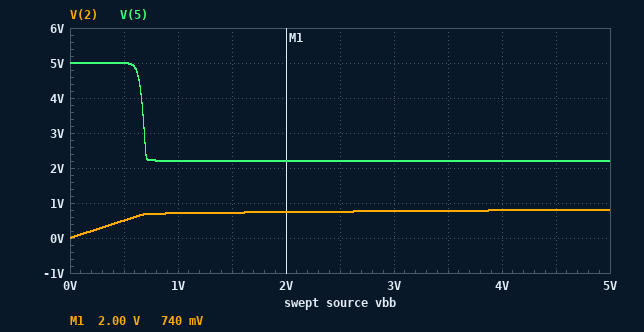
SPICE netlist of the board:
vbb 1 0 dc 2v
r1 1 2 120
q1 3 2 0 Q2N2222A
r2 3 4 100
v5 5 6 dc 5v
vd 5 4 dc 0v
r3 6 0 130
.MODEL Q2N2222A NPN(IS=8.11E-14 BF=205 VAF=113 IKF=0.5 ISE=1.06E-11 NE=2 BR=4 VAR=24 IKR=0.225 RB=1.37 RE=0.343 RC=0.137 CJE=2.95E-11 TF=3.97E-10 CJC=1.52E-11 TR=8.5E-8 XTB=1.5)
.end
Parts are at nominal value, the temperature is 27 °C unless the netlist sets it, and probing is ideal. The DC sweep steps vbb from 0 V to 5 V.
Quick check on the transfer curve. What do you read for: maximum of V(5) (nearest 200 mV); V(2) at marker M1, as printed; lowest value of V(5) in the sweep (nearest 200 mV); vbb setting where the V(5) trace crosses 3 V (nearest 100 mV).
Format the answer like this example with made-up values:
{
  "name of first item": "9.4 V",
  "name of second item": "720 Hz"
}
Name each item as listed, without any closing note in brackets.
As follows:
{
  "maximum of V(5)": "5.0 V",
  "V(2) at marker M1, as printed": "740 mV",
  "lowest value of V(5) in the sweep": "2.2 V",
  "vbb setting where the V(5) trace crosses 3 V": "700 mV"
}
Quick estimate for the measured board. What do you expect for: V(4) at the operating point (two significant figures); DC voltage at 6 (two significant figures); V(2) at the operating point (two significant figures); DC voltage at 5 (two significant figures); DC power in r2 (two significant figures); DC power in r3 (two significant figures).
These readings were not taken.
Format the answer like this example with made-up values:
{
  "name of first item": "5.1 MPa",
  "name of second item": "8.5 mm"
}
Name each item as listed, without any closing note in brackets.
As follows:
{
  "V(4) at the operating point": "2.2 V",
  "DC voltage at 6": "-2.8 V",
  "V(2) at the operating point": "740 mV",
  "DC voltage at 5": "2.2 V",
  "DC power in r2": "47 mW",
  "DC power in r3": "61 mW"
}
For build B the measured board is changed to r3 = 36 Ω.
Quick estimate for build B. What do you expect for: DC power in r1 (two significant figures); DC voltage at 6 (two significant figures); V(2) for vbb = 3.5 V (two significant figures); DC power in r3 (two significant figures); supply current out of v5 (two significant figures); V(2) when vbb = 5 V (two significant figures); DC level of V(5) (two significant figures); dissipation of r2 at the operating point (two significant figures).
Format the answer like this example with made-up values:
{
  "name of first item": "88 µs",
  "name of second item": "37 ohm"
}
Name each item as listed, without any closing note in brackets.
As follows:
{
  "DC power in r1": "13 mW",
  "DC voltage at 6": "-1.3 V",
  "V(2) for vbb = 3.5 V": "790 mV",
  "DC power in r3": "48 mW",
  "supply current out of v5": "36 mA",
  "V(2) when vbb = 5 V": "820 mV",
  "DC level of V(5)": "3.7 V",
  "dissipation of r2 at the operating point": "130 mW"
}
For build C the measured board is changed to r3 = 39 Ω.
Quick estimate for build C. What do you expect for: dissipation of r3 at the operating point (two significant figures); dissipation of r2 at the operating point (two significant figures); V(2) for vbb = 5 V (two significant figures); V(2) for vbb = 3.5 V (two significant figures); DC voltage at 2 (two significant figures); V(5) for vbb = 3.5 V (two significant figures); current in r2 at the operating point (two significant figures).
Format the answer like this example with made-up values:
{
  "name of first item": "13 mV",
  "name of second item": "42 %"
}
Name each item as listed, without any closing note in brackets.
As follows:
{
  "dissipation of r3 at the operating point": "50 mW",
  "dissipation of r2 at the operating point": "130 mW",
  "V(2) for vbb = 5 V": "820 mV",
  "V(2) for vbb = 3.5 V": "790 mV",
  "DC voltage at 2": "750 mV",
  "V(5) for vbb = 3.5 V": "3.6 V",
  "current in r2 at the operating point": "36 mA"
}
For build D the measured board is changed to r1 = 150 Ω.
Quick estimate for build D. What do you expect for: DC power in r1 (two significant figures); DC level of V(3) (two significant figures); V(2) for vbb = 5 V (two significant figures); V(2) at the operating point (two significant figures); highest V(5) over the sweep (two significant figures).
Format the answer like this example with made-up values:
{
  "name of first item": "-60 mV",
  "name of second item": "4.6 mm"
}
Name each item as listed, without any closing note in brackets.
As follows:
{
  "DC power in r1": "11 mW",
  "DC level of V(3)": "33 mV",
  "V(2) for vbb = 5 V": "790 mV",
  "V(2) at the operating point": "730 mV",
  "highest V(5) over the sweep": "5.0 V"
}
